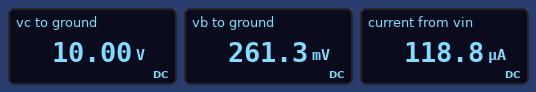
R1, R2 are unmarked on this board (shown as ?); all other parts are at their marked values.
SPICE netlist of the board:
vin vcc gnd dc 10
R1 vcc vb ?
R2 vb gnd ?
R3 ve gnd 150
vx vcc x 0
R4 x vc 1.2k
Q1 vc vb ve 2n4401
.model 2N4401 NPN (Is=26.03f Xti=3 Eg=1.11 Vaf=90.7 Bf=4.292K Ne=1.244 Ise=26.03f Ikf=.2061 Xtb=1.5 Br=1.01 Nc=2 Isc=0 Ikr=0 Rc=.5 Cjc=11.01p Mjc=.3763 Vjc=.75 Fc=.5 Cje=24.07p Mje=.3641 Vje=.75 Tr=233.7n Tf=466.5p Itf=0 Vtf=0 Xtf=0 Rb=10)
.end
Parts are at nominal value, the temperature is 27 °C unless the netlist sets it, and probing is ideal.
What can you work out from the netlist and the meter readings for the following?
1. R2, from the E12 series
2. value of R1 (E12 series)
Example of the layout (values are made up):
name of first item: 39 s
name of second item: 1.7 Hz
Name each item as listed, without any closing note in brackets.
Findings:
R2, from the E12 series: 2.2 kΩ
value of R1: 82 kΩ
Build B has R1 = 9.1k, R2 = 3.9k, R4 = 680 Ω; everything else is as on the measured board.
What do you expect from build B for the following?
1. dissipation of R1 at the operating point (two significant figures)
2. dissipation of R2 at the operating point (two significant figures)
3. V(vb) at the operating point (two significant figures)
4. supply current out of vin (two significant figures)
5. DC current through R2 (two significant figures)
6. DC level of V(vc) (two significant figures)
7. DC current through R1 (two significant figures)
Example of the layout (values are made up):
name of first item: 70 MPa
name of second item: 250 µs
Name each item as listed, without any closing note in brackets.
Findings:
dissipation of R1 at the operating point: 6.2 mW
dissipation of R2 at the operating point: 1.6 mW
V(vb) at the operating point: 2.5 V
supply current out of vin: 13 mA
DC current through R2: 640 µA
DC level of V(vc): 1.9 V
DC current through R1: 820 µA
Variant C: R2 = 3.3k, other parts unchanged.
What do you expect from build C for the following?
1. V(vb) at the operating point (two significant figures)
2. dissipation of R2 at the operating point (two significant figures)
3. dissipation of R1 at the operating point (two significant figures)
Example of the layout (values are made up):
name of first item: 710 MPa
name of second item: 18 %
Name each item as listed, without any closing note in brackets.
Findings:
V(vb) at the operating point: 390 mV
dissipation of R2 at the operating point: 45 µW
dissipation of R1 at the operating point: 1.1 mW
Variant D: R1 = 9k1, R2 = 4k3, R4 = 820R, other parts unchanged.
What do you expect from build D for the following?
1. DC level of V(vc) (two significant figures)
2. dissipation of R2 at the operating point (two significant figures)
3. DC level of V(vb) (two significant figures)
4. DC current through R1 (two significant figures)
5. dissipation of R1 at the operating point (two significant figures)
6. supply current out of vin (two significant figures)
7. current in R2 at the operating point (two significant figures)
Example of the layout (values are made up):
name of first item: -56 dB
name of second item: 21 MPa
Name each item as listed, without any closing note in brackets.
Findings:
DC level of V(vc): 1.7 V
dissipation of R2 at the operating point: 1.2 mW
DC level of V(vb): 2.3 V
DC current through R1: 850 µA
dissipation of R1 at the operating point: 6.6 mW
supply current out of vin: 11 mA
current in R2 at the operating point: 530 µA
